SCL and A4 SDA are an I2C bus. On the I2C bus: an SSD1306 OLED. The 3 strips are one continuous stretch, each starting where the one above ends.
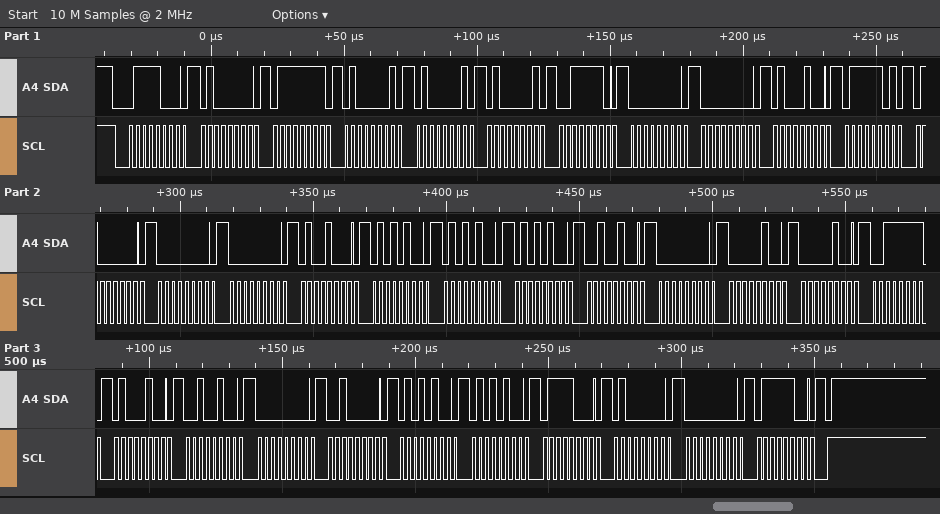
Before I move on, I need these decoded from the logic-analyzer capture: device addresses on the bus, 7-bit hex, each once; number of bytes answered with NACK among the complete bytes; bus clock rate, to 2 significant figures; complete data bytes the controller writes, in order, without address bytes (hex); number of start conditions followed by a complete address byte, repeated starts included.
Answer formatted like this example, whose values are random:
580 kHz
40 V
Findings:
0x3C
0
400 kHz
40 7F 41 41 41 3E 00 00 44 7D 40 00 00 48 54 54 54 24 00 04 04 3F 44 24 00 20 54 54 78 40 00 7C
1
